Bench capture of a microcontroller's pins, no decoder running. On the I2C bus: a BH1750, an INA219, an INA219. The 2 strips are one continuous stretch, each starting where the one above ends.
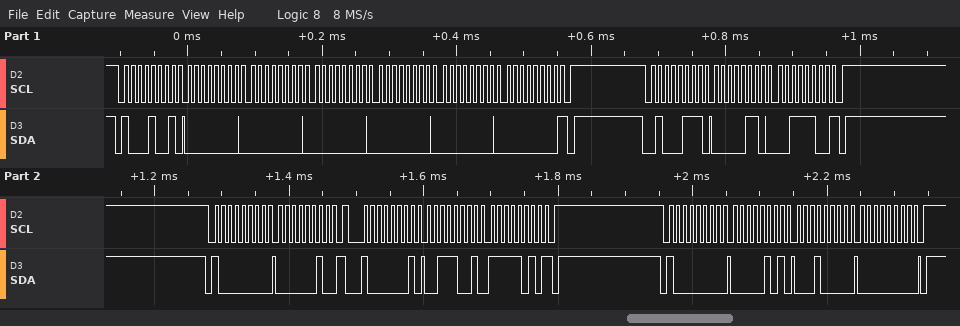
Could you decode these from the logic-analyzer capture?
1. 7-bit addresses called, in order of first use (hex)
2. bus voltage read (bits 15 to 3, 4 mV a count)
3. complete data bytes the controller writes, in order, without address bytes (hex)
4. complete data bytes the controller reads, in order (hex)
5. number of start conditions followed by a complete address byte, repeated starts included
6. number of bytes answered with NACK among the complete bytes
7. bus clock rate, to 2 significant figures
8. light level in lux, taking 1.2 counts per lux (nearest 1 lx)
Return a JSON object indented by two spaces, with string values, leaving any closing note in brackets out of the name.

{
  "7-bit addresses called, in order of first use": "0x44 0x23 0x40",
  "bus voltage read": "7.420 V",
  "complete data bytes the controller writes, in order, without address bytes": "02 05 10 00",
  "complete data bytes the controller reads, in order": "00 00 00 00 00 00 06 3C 39 FA",
  "number of start conditions followed by a complete address byte, repeated starts included": "5",
  "number of bytes answered with NACK among the complete bytes": "3",
  "bus clock rate, to 2 significant figures": "100 kHz",
  "light level in lux, taking 1.2 counts per lux": "1330 lx"
}
